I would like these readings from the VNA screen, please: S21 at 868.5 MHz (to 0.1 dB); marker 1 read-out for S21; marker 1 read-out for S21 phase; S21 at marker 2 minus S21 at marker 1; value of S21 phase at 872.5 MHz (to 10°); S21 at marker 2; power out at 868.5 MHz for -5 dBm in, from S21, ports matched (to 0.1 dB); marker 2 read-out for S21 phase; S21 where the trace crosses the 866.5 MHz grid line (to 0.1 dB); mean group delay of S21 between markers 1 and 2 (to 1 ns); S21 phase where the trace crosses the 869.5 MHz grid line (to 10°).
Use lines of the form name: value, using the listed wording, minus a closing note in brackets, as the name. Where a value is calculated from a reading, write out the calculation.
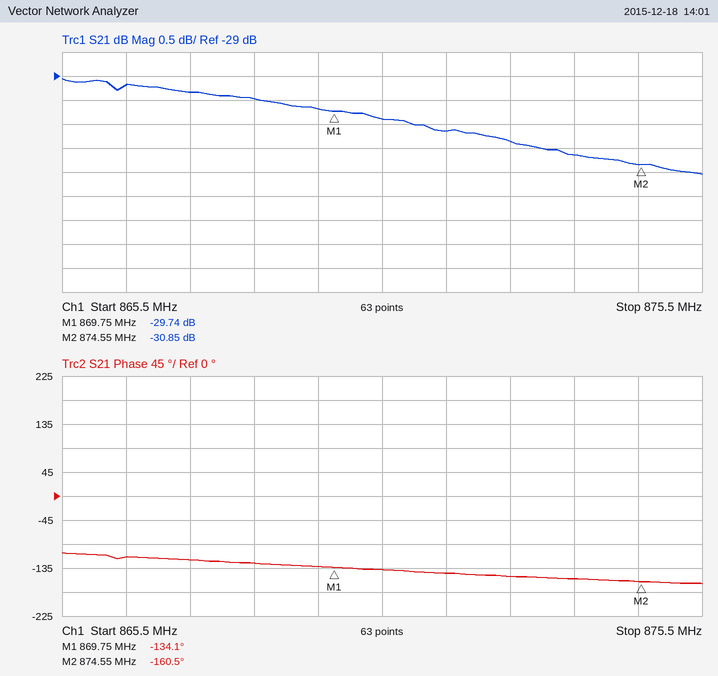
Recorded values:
S21 at 868.5 MHz: -29.5 dB
marker 1 read-out for S21: -29.74 dB
marker 1 read-out for S21 phase: -134.1°
S21 at marker 2 minus S21 at marker 1: -30.85 − (-29.74) = -1.11 dB
value of S21 phase at 872.5 MHz: -150°
S21 at marker 2: -30.85 dB
power out at 868.5 MHz for -5 dBm in, from S21, ports matched: -5 dBm + (-29.5 dB) = -34.5 dBm
marker 2 read-out for S21 phase: -160.5°
S21 where the trace crosses the 866.5 MHz grid line: -29.2 dB
mean group delay of S21 between markers 1 and 2: −(-160.5° − (-134.1°))/(360° × 4.8 MHz) ≈ 15 ns
S21 phase where the trace crosses the 869.5 MHz grid line: -130°
